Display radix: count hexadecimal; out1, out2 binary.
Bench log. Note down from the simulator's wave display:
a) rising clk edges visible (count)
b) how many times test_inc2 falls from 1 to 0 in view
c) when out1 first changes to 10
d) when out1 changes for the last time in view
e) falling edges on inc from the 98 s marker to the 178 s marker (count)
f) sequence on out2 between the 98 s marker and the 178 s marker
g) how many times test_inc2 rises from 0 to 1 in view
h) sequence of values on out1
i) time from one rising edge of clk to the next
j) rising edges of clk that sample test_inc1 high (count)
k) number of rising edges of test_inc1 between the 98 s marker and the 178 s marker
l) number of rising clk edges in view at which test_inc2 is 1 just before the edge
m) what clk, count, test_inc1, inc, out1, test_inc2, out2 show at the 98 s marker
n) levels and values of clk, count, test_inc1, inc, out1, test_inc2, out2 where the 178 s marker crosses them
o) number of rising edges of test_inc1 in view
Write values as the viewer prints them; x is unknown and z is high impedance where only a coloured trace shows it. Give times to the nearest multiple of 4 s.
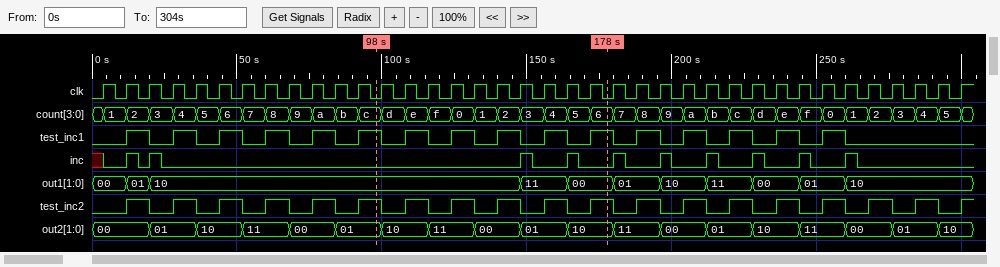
38
18
20 s
260 s
2
01, 10, 11, 00, 01, 10
19
00, 01, 10, 11, 00, 01, 10, 11, 00, 01, 10
8 s
16
5
18
clk=0, count=c, test_inc1=1, inc=0, out1=10, test_inc2=1, out2=01
clk=0, count=6, test_inc1=1, inc=0, out1=00, test_inc2=1, out2=10
16
